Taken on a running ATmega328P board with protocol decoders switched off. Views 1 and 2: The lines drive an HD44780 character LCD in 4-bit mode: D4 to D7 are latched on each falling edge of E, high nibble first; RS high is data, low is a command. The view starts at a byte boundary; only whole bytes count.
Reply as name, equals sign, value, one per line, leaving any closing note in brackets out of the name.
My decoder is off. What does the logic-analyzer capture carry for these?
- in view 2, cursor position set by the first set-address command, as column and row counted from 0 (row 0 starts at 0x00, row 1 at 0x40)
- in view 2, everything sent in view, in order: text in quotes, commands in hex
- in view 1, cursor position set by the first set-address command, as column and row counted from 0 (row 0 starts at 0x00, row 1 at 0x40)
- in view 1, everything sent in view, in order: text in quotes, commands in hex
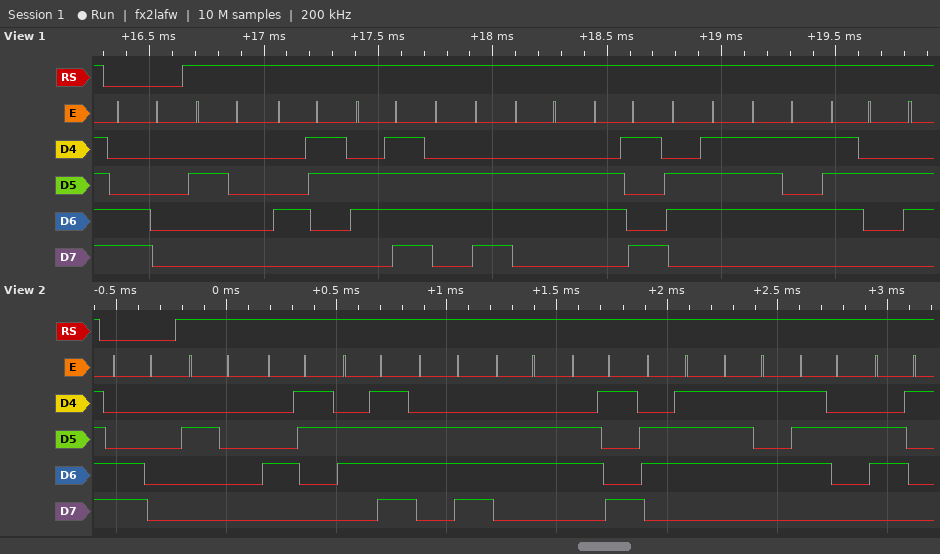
in view 2, cursor position set by the first set-address command, as column and row counted from 0 = column 0, row 1
in view 2, everything sent in view, in order: text in quotes, commands in hex = 0xC0 " Configura"
in view 1, cursor position set by the first set-address command, as column and row counted from 0 = column 0, row 1
in view 1, everything sent in view, in order: text in quotes, commands in hex = 0xC0 " Configur"
